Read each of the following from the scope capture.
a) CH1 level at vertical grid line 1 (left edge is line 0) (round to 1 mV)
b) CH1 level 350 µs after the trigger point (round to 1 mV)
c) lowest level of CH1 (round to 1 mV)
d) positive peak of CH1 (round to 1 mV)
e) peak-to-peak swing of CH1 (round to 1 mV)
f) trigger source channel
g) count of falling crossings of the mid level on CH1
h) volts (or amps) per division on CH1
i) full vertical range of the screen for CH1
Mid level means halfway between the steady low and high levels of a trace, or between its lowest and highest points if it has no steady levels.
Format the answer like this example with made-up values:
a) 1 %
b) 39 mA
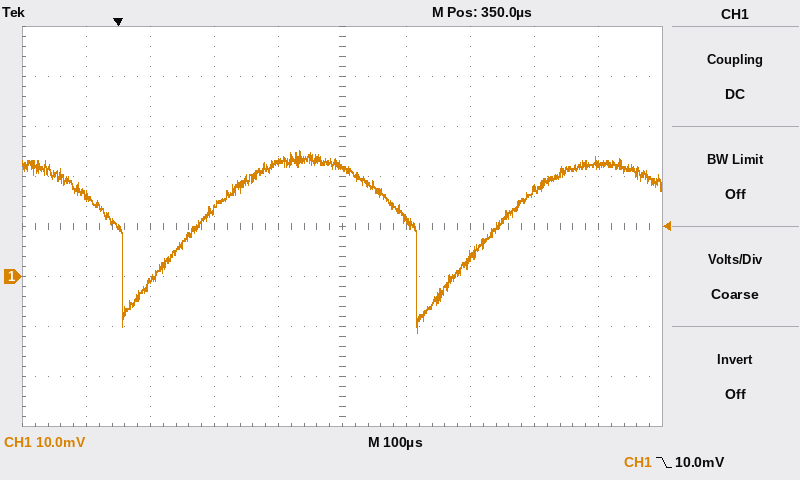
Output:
a) 16 mV
b) 22 mV
c) -11 mV
d) 25 mV
e) 36 mV
f) CH1
g) 2
h) 10 mV
i) 80 mV
